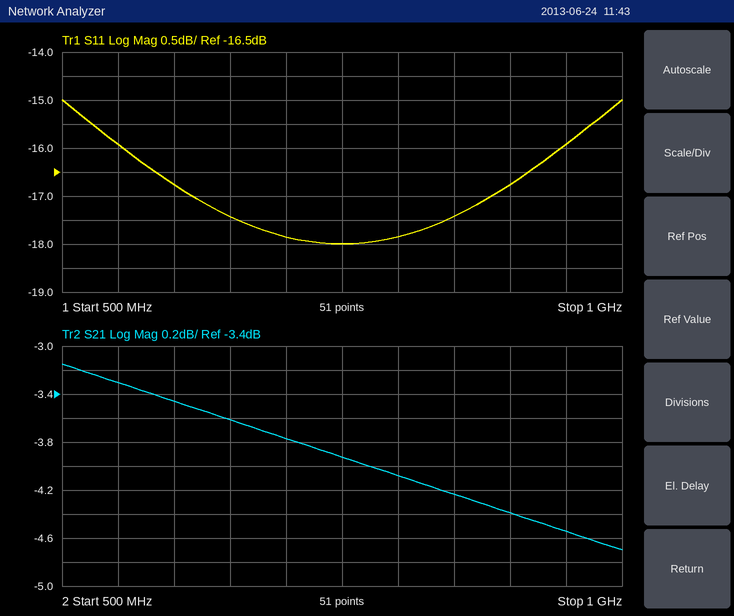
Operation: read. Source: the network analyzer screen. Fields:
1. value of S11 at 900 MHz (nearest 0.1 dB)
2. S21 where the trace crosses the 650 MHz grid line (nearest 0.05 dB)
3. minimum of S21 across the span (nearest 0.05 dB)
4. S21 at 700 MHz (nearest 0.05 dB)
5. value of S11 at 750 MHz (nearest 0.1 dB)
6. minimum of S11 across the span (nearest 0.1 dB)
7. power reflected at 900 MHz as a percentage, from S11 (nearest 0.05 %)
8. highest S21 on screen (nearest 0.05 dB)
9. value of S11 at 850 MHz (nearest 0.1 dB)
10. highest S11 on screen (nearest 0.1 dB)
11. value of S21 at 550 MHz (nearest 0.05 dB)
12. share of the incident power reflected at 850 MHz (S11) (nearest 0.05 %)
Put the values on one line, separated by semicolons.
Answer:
-16.8 dB; -3.60 dB; -4.70 dB; -3.75 dB; -18.0 dB; -18.0 dB; 2.10 %; -3.15 dB; -17.4 dB; -15.0 dB; -3.30 dB; 1.80 %
